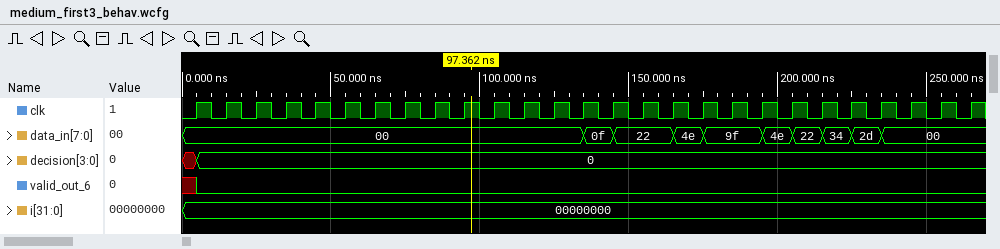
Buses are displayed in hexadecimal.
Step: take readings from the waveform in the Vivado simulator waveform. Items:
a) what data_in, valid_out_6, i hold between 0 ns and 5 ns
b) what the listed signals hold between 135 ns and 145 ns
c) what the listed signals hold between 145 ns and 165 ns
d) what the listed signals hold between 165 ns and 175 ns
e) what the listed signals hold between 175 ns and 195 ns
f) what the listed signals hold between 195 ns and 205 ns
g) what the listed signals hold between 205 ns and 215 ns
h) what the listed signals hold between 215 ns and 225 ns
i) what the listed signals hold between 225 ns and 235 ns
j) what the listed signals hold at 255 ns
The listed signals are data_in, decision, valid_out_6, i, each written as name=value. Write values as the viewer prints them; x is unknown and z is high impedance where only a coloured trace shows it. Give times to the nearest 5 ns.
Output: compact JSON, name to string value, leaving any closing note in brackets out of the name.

{"what data_in, valid_out_6, i hold between 0 ns and 5 ns": "data_in=00, valid_out_6=x, i=00000000", "what the listed signals hold between 135 ns and 145 ns": "data_in=0f, decision=0, valid_out_6=0, i=00000000", "what the listed signals hold between 145 ns and 165 ns": "data_in=22, decision=0, valid_out_6=0, i=00000000", "what the listed signals hold between 165 ns and 175 ns": "data_in=4e, decision=0, valid_out_6=0, i=00000000", "what the listed signals hold between 175 ns and 195 ns": "data_in=9f, decision=0, valid_out_6=0, i=00000000", "what the listed signals hold between 195 ns and 205 ns": "data_in=4e, decision=0, valid_out_6=0, i=00000000", "what the listed signals hold between 205 ns and 215 ns": "data_in=22, decision=0, valid_out_6=0, i=00000000", "what the listed signals hold between 215 ns and 225 ns": "data_in=34, decision=0, valid_out_6=0, i=00000000", "what the listed signals hold between 225 ns and 235 ns": "data_in=2d, decision=0, valid_out_6=0, i=00000000", "what the listed signals hold at 255 ns": "data_in=00, decision=0, valid_out_6=0, i=00000000"}
